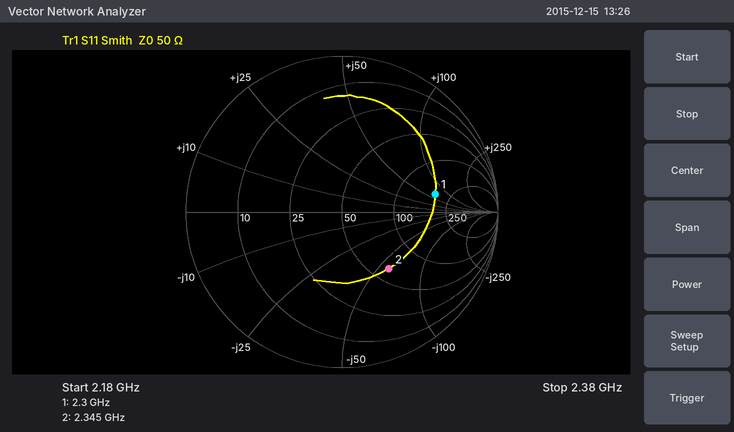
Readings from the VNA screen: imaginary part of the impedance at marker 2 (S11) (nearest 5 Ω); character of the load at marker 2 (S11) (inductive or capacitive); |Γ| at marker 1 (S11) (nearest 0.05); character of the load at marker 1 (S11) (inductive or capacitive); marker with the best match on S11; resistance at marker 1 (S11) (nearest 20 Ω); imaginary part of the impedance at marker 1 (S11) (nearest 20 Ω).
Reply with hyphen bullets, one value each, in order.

- -60 Ω
- capacitive
- 0.60
- inductive
- marker 2
- 180 Ω
- +60 Ω
